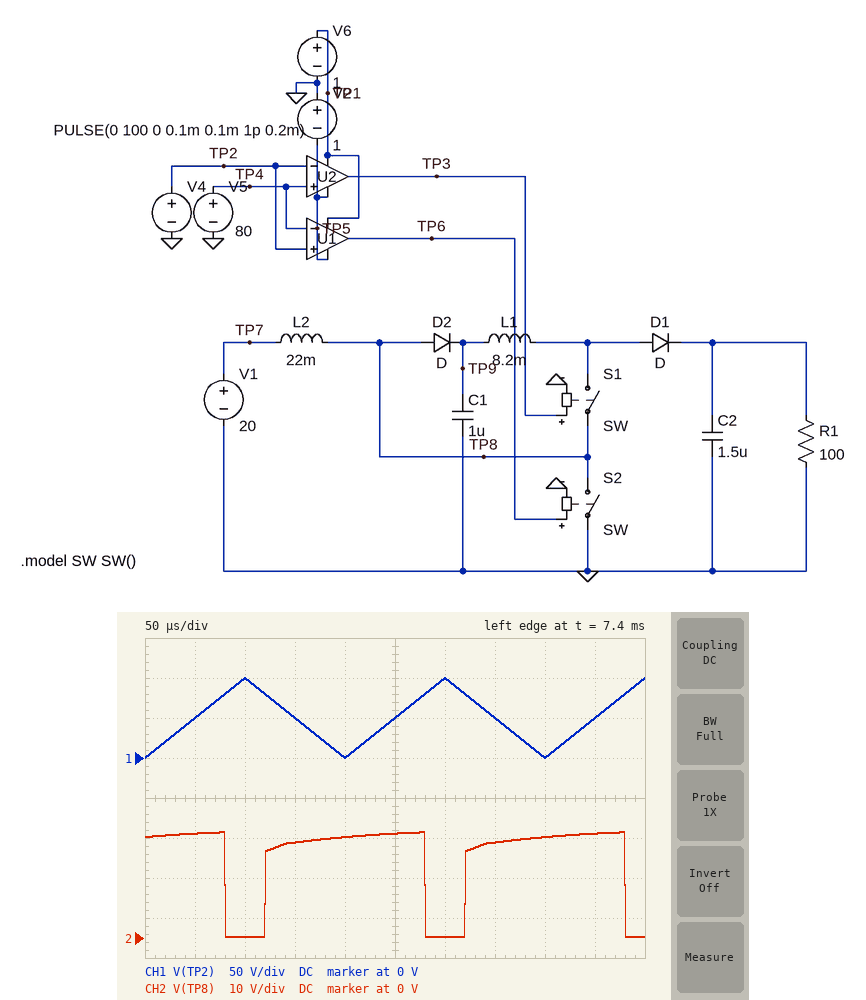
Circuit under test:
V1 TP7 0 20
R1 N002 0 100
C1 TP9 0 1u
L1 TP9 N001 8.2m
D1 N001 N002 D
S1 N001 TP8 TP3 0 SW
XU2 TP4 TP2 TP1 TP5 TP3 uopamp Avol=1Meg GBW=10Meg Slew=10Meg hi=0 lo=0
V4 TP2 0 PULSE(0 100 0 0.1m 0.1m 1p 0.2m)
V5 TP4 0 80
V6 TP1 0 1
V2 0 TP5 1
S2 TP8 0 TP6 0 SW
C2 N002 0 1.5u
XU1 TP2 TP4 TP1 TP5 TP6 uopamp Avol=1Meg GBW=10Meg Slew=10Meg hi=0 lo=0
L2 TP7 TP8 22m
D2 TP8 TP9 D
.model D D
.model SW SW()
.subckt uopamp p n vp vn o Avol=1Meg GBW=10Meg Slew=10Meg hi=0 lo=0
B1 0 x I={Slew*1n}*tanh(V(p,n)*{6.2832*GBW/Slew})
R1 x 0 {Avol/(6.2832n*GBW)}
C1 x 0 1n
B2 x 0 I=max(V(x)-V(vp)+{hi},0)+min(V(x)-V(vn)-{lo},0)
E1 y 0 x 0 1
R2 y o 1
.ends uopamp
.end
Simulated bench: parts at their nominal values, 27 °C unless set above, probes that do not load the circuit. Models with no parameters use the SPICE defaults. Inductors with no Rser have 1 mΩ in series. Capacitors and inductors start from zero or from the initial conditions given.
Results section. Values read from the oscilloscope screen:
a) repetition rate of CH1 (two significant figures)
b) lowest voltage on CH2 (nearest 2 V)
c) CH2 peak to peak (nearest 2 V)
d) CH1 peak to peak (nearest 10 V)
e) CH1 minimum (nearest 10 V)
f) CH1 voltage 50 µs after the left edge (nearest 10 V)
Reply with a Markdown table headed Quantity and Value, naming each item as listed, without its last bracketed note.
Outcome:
| Quantity | Value |
|---|---|
| repetition rate of CH1 | 5.0 kHz |
| lowest voltage on CH2 | 0 V |
| CH2 peak to peak | 26 V |
| CH1 peak to peak | 100 V |
| CH1 minimum | 0 V |
| CH1 voltage 50 µs after the left edge | 50 V |
